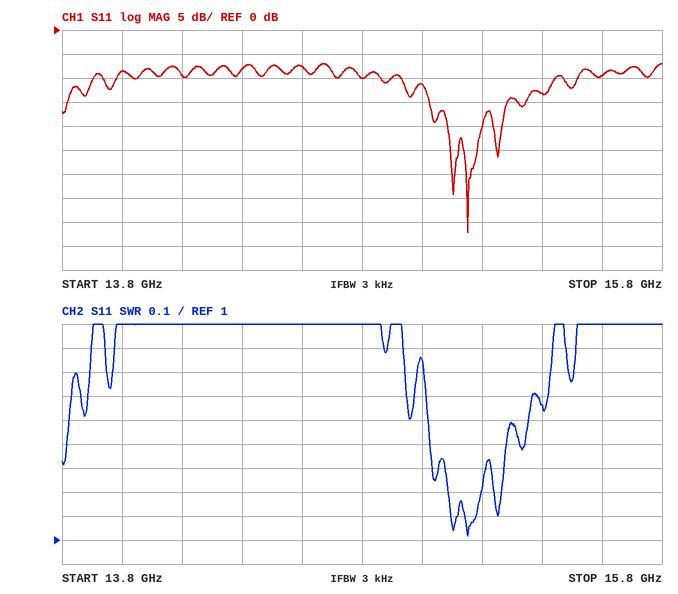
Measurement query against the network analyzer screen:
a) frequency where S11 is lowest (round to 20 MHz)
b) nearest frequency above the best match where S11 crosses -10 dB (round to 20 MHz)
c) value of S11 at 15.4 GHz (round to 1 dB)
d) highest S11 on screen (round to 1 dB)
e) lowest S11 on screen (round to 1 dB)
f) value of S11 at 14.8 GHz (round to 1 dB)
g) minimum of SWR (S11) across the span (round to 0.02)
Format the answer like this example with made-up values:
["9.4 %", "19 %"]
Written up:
["15.16 GHz", "15.44 GHz", "-13 dB", "-7 dB", "-42 dB", "-10 dB", "1.02"]
